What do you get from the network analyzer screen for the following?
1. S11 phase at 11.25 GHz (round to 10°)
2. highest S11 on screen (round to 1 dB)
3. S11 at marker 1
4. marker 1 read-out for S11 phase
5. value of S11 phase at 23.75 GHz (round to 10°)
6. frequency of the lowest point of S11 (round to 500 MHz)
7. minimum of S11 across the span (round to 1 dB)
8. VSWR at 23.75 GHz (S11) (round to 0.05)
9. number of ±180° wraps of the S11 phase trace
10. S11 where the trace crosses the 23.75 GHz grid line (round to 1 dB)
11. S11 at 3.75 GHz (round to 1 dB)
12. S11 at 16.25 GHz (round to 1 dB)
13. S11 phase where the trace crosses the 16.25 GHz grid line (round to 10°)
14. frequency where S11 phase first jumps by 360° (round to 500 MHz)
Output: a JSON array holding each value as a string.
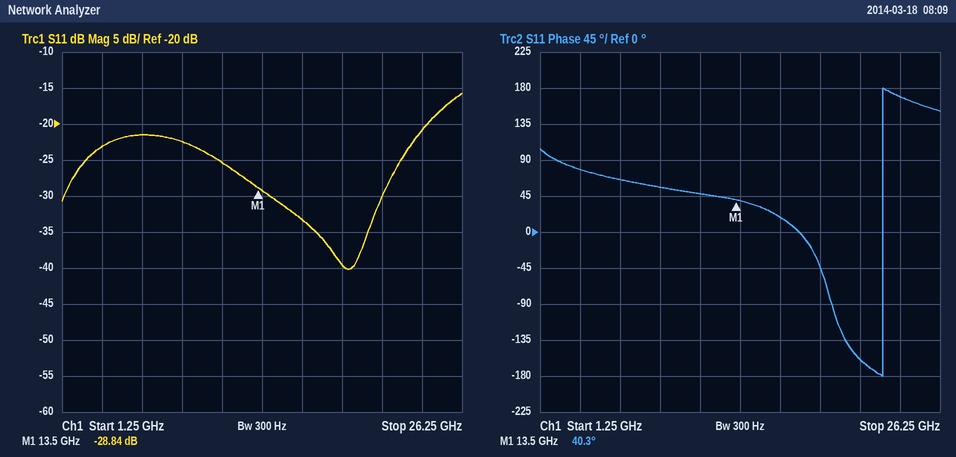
["50°", "-16 dB", "-28.84 dB", "40.3°", "170°", "19.0 GHz", "-40 dB", "1.20", "1", "-21 dB", "-23 dB", "-33 dB", "20°", "22.5 GHz"]
